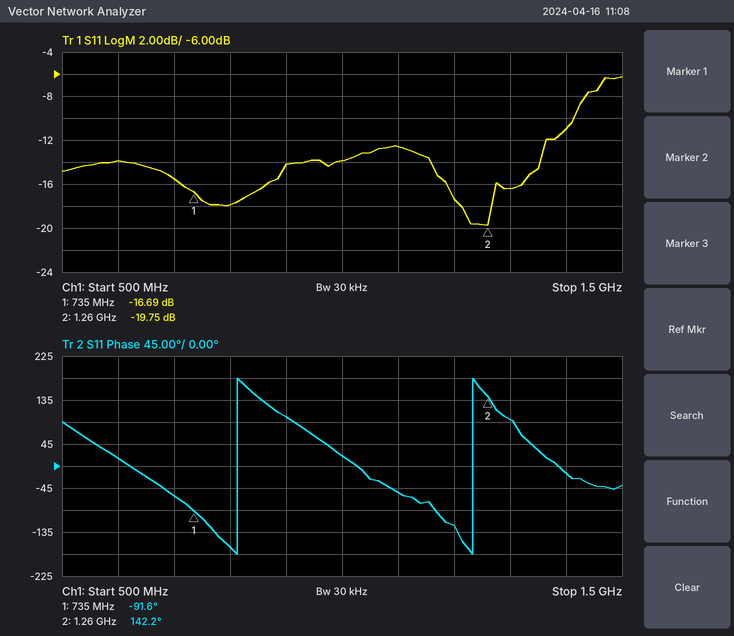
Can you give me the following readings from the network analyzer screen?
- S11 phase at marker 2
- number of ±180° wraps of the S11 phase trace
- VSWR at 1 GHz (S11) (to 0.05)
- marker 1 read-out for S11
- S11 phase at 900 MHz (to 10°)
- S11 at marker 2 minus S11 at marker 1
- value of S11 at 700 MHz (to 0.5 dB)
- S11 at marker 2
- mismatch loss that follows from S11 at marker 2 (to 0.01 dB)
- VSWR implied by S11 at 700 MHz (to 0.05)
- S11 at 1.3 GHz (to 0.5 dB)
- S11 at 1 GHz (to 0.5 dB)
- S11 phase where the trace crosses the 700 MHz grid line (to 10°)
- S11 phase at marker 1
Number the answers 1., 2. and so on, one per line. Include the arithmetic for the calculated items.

1. 142.2°
2. 2
3. |Γ| = 10^(-14/20) = 0.1995; VSWR = (1 + 0.1995)/(1 − 0.1995) ≈ 1.50
4. -16.69 dB
5. 100°
6. -19.75 − (-16.69) = -3.06 dB
7. -15.5 dB
8. -19.75 dB
9. −10 log10(1 − 10^(-19.75/10)) ≈ 0.05 dB
10. |Γ| = 10^(-15.5/20) = 0.1679; VSWR = (1 + 0.1679)/(1 − 0.1679) ≈ 1.40
11. -16.5 dB
12. -14.0 dB
13. -60°
14. -91.6°
